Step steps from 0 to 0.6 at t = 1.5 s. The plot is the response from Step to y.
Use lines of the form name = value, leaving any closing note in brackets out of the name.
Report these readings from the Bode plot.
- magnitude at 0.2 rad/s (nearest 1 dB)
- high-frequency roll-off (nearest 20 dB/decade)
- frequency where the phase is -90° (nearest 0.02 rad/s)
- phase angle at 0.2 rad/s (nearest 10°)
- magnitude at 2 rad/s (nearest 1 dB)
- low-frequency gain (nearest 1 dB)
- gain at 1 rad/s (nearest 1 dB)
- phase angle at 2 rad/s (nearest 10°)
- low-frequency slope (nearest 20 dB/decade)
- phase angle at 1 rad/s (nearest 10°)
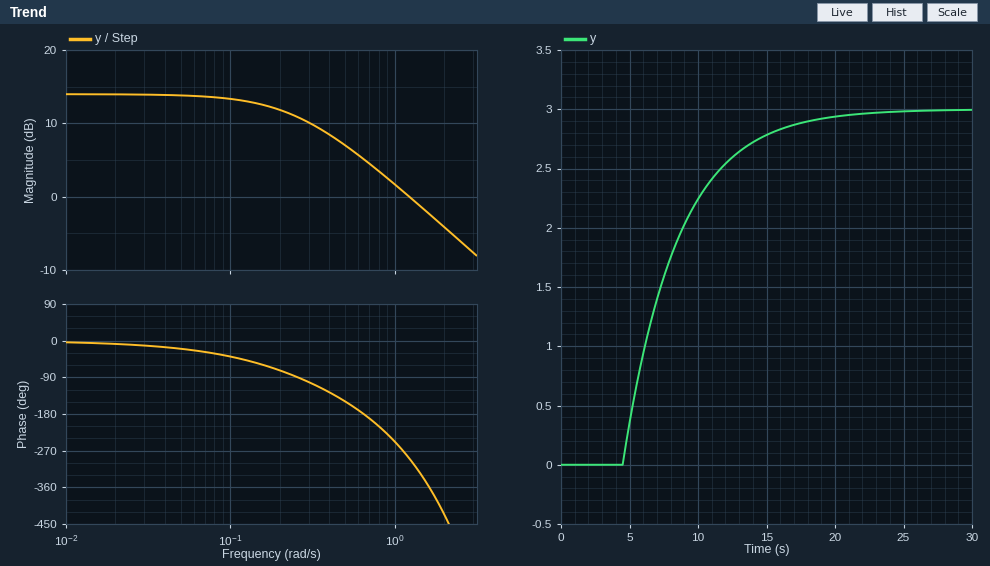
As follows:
magnitude at 0.2 rad/s = 12 dB
high-frequency roll-off = -20 dB/decade
frequency where the phase is -90° = 0.26 rad/s
phase angle at 0.2 rad/s = -70°
magnitude at 2 rad/s = -4 dB
low-frequency gain = 14 dB
gain at 1 rad/s = 2 dB
phase angle at 2 rad/s = -430°
low-frequency slope = 0 dB/decade
phase angle at 1 rad/s = -250°
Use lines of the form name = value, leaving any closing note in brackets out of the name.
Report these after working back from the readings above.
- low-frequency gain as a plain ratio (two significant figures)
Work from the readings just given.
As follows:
low-frequency gain as a plain ratio = 5.0
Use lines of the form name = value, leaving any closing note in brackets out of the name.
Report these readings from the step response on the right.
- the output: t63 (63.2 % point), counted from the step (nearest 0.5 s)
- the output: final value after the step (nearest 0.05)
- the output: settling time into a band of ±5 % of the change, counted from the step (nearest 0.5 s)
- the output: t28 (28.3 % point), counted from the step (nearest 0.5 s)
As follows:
the output: t63 (63.2 % point), counted from the step = 7.0 s
the output: final value after the step = 3.00
the output: settling time into a band of ±5 % of the change, counted from the step = 15.0 s
the output: t28 (28.3 % point), counted from the step = 4.5 s
